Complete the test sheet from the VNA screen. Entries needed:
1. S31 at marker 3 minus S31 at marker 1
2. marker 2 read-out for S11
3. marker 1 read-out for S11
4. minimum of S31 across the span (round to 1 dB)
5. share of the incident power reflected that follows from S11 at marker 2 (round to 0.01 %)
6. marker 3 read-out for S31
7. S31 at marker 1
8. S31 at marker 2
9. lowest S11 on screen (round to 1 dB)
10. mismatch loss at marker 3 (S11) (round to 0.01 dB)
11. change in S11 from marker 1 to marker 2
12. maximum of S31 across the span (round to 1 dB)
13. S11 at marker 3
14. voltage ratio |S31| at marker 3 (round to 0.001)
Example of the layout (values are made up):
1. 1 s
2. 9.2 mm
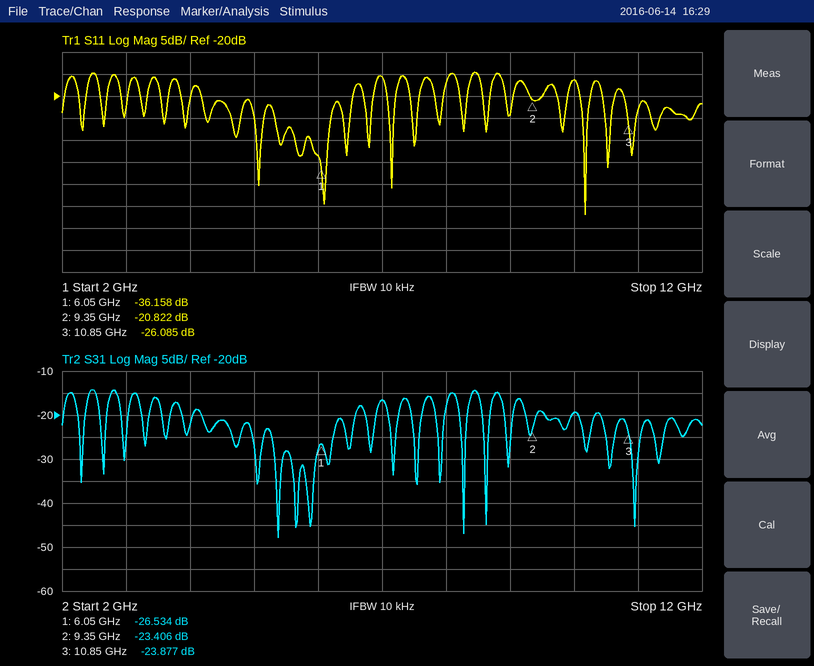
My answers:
1. 2.657 dB
2. -20.822 dB
3. -36.158 dB
4. -48 dB
5. 0.83 %
6. -23.877 dB
7. -26.534 dB
8. -23.406 dB
9. -47 dB
10. 0.01 dB
11. 15.336 dB
12. -14 dB
13. -26.085 dB
14. 0.064
